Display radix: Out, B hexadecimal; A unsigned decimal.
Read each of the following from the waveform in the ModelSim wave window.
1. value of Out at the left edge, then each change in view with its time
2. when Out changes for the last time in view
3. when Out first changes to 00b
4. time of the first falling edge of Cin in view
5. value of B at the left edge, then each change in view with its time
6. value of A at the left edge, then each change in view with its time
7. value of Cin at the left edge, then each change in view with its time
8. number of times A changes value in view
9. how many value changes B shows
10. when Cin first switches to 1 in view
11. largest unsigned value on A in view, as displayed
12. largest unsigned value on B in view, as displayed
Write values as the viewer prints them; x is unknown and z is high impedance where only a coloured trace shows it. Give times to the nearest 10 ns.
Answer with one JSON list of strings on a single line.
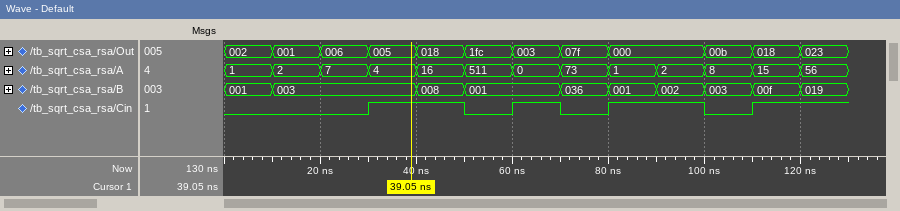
["002, 001 at 10 ns, 006 at 20 ns, 005 at 30 ns, 018 at 40 ns, 1fc at 50 ns, 003 at 60 ns, 07f at 70 ns, 000 at 80 ns, 00b at 100 ns, 018 at 110 ns, 023 at 120 ns", "120 ns", "100 ns", "50 ns", "001, 003 at 10 ns, 008 at 40 ns, 001 at 50 ns, 036 at 70 ns, 001 at 80 ns, 002 at 90 ns, 003 at 100 ns, 00f at 110 ns, 019 at 120 ns", "1, 2 at 10 ns, 7 at 20 ns, 4 at 30 ns, 16 at 40 ns, 511 at 50 ns, 0 at 60 ns, 73 at 70 ns, 1 at 80 ns, 2 at 90 ns, 8 at 100 ns, 15 at 110 ns, 56 at 120 ns", "0, 1 at 30 ns, 0 at 50 ns, 1 at 60 ns, 0 at 70 ns, 1 at 80 ns, 0 at 100 ns, 1 at 110 ns", "12", "9", "30 ns", "511", "036"]
